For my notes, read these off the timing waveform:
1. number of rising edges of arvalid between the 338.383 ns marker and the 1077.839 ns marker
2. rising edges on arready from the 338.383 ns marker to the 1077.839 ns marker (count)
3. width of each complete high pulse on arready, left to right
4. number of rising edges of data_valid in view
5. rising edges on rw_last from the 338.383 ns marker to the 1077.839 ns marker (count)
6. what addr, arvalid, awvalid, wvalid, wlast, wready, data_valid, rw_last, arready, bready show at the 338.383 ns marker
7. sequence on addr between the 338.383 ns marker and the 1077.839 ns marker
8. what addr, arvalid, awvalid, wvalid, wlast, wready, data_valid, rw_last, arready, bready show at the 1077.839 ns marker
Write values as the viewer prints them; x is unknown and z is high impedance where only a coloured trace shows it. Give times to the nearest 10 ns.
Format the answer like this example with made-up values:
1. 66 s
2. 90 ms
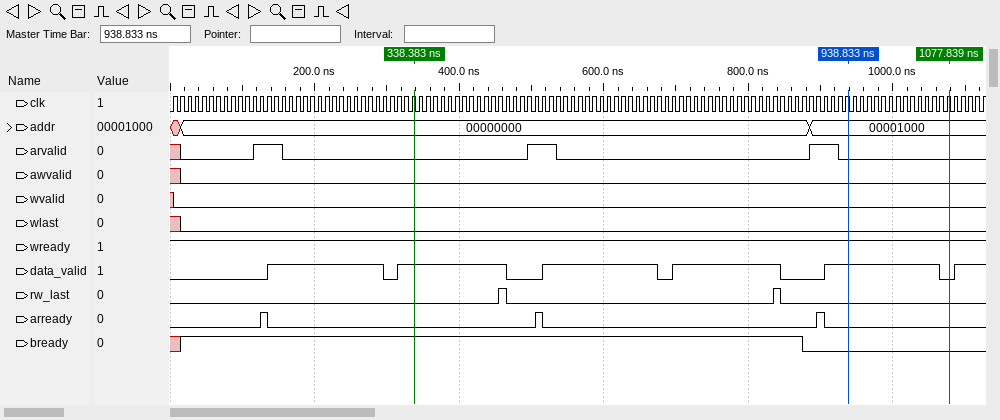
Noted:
1. 2
2. 2
3. 10 ns, 10 ns, 10 ns
4. 6
5. 2
6. addr=00000000, arvalid=0, awvalid=0, wvalid=0, wlast=0, wready=1, data_valid=1, rw_last=0, arready=0, bready=1
7. 00000000, 00001000
8. addr=00001000, arvalid=0, awvalid=0, wvalid=0, wlast=0, wready=1, data_valid=0, rw_last=0, arready=0, bready=0
